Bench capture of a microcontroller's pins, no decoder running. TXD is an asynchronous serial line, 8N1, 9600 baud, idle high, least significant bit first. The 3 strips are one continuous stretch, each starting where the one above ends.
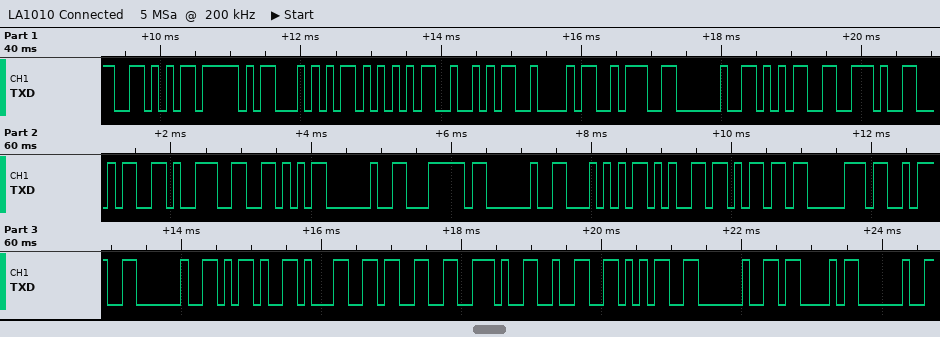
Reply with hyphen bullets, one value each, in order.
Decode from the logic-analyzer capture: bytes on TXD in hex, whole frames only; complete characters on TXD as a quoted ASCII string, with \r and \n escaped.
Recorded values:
- 56 5F 54 55 52 42 3A 20 35 2E 34 39 56 20 7C 20 54 65 6D 70 3A 20 2D 31 33 2E 32 35 20 43 20
- "V_TURB: 5.49V | Temp: -13.25 C "
